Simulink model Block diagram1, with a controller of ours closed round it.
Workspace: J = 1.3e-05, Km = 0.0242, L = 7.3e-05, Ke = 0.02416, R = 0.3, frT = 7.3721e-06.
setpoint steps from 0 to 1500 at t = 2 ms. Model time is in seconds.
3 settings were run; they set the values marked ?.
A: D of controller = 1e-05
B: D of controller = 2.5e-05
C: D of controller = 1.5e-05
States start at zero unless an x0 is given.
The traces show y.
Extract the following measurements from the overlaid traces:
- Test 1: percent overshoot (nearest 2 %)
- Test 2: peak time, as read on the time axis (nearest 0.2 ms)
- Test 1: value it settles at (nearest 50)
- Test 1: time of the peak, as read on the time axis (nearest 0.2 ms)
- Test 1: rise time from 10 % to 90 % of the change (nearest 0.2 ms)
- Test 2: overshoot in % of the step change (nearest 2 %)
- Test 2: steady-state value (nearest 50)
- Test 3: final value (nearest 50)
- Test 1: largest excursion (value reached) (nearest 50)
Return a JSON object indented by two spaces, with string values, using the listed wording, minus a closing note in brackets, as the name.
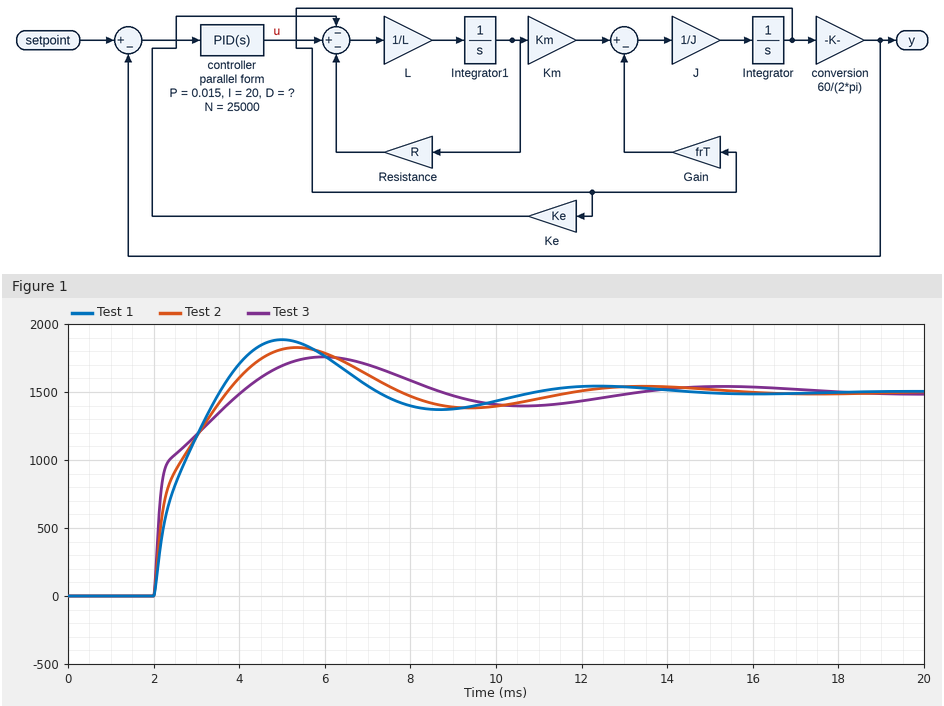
{
  "Test 1: percent overshoot": "26 %",
  "Test 2: peak time, as read on the time axis": "5.4 ms",
  "Test 1: value it settles at": "1500",
  "Test 1: time of the peak, as read on the time axis": "5.0 ms",
  "Test 1: rise time from 10 % to 90 % of the change": "1.2 ms",
  "Test 2: overshoot in % of the step change": "22 %",
  "Test 2: steady-state value": "1500",
  "Test 3: final value": "1500",
  "Test 1: largest excursion (value reached)": "1900"
}
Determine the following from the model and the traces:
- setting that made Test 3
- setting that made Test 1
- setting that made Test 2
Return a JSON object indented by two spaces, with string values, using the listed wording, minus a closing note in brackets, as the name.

{
  "setting that made Test 3": "B",
  "setting that made Test 1": "A",
  "setting that made Test 2": "C"
}
